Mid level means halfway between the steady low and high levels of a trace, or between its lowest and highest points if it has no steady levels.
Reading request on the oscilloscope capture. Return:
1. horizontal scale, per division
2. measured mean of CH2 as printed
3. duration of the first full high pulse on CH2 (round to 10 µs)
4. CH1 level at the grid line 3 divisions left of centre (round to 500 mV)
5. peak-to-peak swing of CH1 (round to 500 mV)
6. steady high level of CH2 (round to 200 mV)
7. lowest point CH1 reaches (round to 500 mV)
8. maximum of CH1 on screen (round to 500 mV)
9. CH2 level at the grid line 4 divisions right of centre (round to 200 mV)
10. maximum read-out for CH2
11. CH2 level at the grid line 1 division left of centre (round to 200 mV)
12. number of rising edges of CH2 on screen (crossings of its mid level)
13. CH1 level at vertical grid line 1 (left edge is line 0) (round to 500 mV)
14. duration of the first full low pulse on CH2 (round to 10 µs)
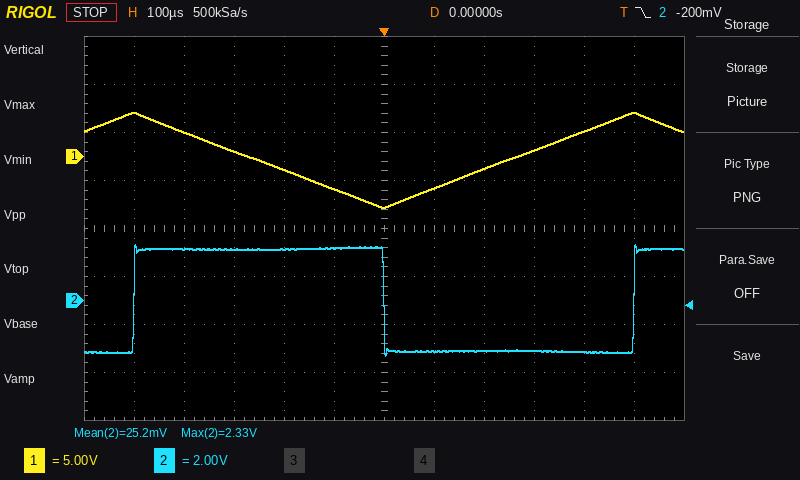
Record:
100 µs
25.2 mV
500 µs
500 mV
10.0 V
2.2 V
-5.5 V
4.5 V
-2.2 V
2.33 V
2.2 V
2
4.5 V
500 µs
